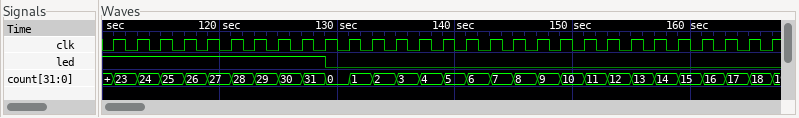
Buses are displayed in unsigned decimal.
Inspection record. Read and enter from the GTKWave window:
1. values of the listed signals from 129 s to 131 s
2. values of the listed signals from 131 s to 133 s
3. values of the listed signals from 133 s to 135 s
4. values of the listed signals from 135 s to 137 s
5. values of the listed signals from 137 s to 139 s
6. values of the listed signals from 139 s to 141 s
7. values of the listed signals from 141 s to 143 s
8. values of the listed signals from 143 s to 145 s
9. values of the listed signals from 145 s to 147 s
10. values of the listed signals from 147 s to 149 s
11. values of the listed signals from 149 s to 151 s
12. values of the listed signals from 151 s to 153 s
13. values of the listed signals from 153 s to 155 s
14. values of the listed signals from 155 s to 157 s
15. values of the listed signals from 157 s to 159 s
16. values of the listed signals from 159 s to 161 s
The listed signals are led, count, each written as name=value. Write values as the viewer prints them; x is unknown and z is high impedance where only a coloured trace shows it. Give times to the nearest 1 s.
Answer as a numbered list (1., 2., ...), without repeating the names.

1. led=0, count=0
2. led=0, count=1
3. led=0, count=2
4. led=0, count=3
5. led=0, count=4
6. led=0, count=5
7. led=0, count=6
8. led=0, count=7
9. led=0, count=8
10. led=0, count=9
11. led=0, count=10
12. led=0, count=11
13. led=0, count=12
14. led=0, count=13
15. led=0, count=14
16. led=0, count=15
